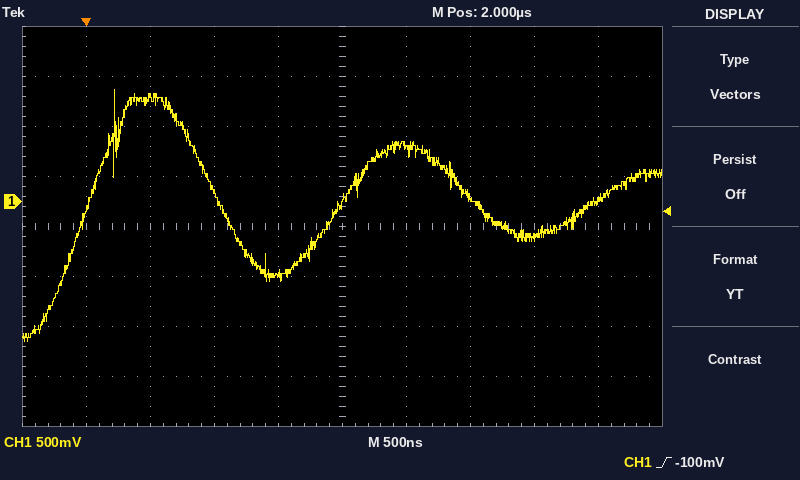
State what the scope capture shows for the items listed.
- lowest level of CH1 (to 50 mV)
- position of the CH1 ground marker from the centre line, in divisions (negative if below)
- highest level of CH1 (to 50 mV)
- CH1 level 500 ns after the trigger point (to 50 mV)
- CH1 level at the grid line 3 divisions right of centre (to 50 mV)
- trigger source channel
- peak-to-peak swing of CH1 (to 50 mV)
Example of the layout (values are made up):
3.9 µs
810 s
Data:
-1.40 V
+0.5 div
1.10 V
1.05 V
-350 mV
CH1
2.50 V
